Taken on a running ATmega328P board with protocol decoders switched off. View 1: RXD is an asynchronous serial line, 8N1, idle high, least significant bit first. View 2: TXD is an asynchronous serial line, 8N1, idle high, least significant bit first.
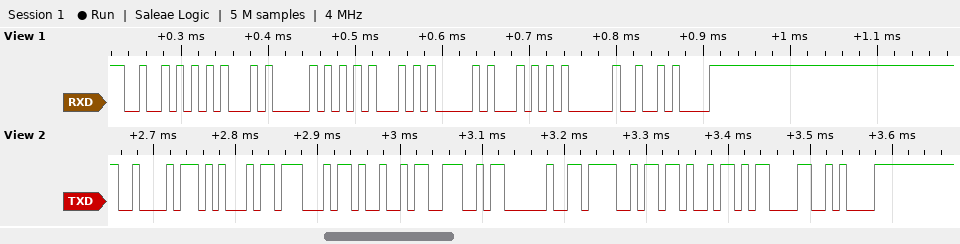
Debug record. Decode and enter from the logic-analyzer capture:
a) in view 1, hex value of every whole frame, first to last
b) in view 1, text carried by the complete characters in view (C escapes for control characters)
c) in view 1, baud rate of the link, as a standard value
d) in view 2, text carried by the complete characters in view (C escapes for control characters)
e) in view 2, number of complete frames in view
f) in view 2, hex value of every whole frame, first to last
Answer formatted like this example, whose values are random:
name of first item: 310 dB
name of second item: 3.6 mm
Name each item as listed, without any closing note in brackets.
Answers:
in view 1, hex value of every whole frame, first to last: 52 45 50 45 41 54 20 0A
in view 1, text carried by the complete characters in view: "REPEAT \n"
in view 1, baud rate of the link, as a standard value: 115200 baud
in view 2, text carried by the complete characters in view: "BEGIN OK\r\n"
in view 2, number of complete frames in view: 10
in view 2, hex value of every whole frame, first to last: 42 45 47 49 4E 20 4F 4B 0D 0A
